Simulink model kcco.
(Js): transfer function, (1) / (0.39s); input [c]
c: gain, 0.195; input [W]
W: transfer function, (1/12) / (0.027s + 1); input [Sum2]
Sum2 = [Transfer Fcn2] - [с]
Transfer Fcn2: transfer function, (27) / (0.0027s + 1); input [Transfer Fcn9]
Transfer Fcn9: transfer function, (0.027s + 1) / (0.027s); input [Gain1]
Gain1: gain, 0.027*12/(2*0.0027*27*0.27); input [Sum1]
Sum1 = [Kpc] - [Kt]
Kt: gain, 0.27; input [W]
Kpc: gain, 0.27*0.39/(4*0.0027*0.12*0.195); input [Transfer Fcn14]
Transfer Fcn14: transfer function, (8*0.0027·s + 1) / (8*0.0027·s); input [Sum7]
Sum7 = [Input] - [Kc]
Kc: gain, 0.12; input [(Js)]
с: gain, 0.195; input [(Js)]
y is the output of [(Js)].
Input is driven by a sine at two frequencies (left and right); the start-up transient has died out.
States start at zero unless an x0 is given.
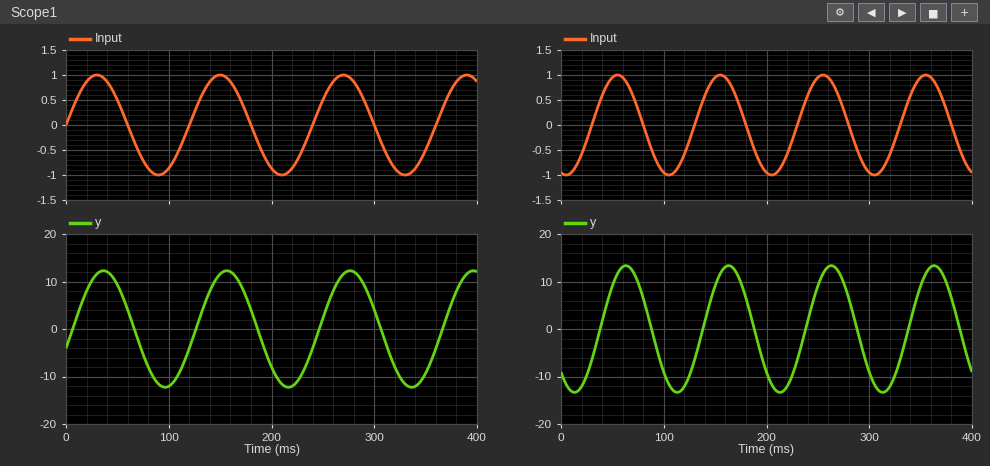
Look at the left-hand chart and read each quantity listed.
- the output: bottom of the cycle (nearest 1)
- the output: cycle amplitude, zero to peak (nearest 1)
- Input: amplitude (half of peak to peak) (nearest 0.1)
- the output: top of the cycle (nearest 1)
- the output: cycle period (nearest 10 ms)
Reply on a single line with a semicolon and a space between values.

-12; 12; 1.0; 12; 120 ms
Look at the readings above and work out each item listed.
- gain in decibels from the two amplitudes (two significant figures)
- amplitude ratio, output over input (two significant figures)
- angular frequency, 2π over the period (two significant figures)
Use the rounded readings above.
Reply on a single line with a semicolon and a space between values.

22 dB; 12; 0.052 rad/ms
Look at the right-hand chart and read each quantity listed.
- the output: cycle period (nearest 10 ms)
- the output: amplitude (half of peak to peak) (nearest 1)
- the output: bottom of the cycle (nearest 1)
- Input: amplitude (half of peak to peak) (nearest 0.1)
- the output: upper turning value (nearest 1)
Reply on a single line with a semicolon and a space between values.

100 ms; 13; -13; 1.0; 13
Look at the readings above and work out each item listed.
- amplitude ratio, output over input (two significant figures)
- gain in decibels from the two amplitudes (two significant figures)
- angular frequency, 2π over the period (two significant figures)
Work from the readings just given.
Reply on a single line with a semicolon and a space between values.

13; 22 dB; 0.063 rad/ms
